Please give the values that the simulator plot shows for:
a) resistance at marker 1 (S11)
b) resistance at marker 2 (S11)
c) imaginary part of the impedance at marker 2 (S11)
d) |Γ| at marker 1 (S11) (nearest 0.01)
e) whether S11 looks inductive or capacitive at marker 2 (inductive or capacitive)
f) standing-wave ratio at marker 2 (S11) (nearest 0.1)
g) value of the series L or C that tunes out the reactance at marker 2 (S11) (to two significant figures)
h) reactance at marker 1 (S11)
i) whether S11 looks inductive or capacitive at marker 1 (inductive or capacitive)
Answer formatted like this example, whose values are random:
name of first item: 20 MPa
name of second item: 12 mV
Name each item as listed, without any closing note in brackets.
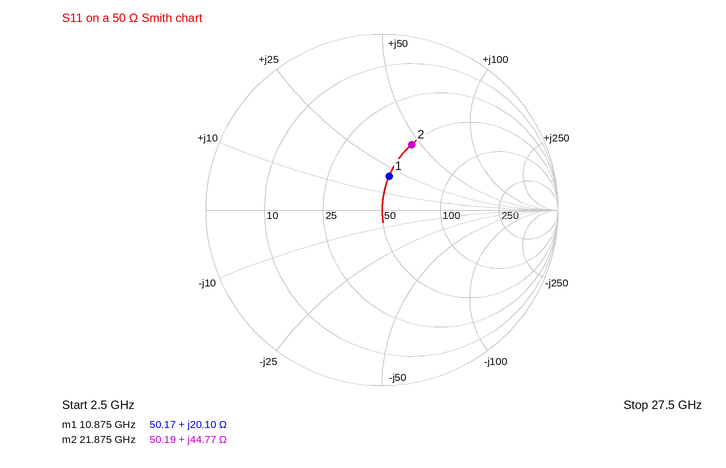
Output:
resistance at marker 1: 50.17 Ω
resistance at marker 2: 50.19 Ω
imaginary part of the impedance at marker 2: +44.77 Ω
|Γ| at marker 1 (S11): 0.20
whether S11 looks inductive or capacitive at marker 2: inductive
standing-wave ratio at marker 2 (S11): 2.4
value of the series L or C that tunes out the reactance at marker 2 (S11): 160 fF
reactance at marker 1: +20.10 Ω
whether S11 looks inductive or capacitive at marker 1: inductive
